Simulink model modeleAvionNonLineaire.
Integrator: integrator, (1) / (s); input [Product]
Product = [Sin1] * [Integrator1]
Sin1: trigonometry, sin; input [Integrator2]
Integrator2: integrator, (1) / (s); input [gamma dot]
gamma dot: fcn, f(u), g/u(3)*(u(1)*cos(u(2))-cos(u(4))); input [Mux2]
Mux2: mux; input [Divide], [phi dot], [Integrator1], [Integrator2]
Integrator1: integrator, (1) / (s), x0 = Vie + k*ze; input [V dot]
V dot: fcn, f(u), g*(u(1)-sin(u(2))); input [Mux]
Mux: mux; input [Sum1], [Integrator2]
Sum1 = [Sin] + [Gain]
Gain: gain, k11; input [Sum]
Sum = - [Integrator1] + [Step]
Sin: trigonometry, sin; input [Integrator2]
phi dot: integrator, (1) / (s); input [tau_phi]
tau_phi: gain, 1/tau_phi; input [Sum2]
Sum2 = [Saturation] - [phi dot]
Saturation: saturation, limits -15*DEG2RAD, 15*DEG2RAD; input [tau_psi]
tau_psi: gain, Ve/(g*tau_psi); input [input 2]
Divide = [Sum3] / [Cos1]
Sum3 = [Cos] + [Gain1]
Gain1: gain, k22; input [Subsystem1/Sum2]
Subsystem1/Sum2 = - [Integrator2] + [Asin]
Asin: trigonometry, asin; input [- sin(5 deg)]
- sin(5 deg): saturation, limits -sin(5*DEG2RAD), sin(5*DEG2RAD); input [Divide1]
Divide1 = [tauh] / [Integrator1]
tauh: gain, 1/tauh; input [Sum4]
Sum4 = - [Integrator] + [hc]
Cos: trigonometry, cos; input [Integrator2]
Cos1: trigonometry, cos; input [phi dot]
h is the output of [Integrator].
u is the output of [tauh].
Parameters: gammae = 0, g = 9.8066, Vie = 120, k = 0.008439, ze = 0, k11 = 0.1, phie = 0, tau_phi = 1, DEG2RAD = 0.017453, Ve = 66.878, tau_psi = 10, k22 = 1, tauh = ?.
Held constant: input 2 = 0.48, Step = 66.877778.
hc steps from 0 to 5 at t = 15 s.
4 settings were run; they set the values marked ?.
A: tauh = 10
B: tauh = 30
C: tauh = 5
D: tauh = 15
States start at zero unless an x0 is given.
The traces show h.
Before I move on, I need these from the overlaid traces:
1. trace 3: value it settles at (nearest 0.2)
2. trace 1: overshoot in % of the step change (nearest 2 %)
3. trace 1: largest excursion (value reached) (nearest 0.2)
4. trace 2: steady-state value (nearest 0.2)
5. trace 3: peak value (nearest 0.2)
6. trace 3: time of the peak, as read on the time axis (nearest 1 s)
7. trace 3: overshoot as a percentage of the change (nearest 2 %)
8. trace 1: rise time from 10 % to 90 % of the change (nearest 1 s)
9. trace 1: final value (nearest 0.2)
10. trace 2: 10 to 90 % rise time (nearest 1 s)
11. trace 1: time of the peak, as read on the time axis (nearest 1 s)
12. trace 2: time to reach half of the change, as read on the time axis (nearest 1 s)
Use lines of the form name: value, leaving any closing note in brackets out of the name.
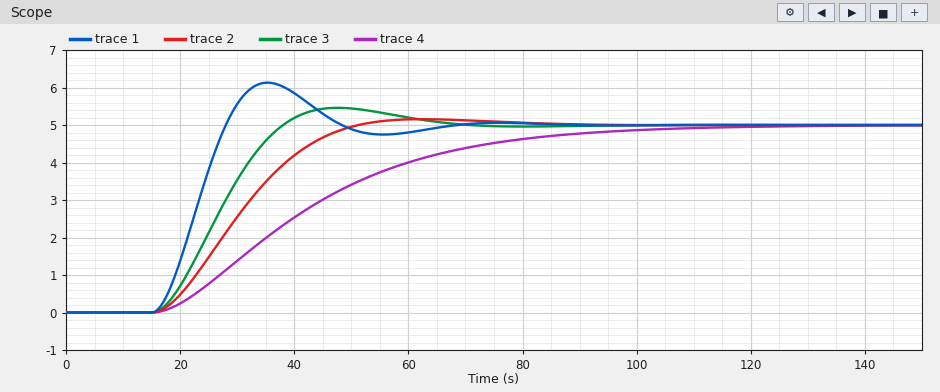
trace 3: value it settles at: 5.0
trace 1: overshoot in % of the step change: 22 %
trace 1: largest excursion (value reached): 6.2
trace 2: steady-state value: 5.0
trace 3: peak value: 5.4
trace 3: time of the peak, as read on the time axis: 48 s
trace 3: overshoot as a percentage of the change: 10 %
trace 1: rise time from 10 % to 90 % of the change: 9 s
trace 1: final value: 5.0
trace 2: 10 to 90 % rise time: 23 s
trace 1: time of the peak, as read on the time axis: 35 s
trace 2: time to reach half of the change, as read on the time axis: 30 s
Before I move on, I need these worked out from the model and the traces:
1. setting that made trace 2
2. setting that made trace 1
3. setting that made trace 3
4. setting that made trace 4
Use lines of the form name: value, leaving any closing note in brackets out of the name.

setting that made trace 2: D
setting that made trace 1: C
setting that made trace 3: A
setting that made trace 4: B
